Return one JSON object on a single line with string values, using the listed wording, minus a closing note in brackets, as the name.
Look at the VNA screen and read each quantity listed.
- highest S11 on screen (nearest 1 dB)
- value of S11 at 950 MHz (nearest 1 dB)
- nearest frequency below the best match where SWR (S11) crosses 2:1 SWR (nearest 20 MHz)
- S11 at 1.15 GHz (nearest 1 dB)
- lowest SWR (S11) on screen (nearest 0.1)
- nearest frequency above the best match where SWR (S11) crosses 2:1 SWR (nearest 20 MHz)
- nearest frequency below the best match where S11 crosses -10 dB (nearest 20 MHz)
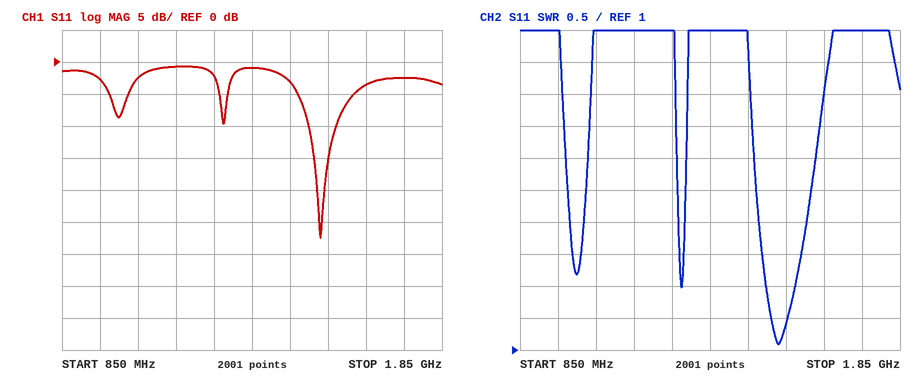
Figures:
{"highest S11 on screen": "-1 dB", "value of S11 at 950 MHz": "-3 dB", "nearest frequency below the best match where SWR (S11) crosses 2:1 SWR": "1.50 GHz", "S11 at 1.15 GHz": "-1 dB", "lowest SWR (S11) on screen": "1.1", "nearest frequency above the best match where SWR (S11) crosses 2:1 SWR": "1.58 GHz", "nearest frequency below the best match where S11 crosses -10 dB": "1.50 GHz"}
